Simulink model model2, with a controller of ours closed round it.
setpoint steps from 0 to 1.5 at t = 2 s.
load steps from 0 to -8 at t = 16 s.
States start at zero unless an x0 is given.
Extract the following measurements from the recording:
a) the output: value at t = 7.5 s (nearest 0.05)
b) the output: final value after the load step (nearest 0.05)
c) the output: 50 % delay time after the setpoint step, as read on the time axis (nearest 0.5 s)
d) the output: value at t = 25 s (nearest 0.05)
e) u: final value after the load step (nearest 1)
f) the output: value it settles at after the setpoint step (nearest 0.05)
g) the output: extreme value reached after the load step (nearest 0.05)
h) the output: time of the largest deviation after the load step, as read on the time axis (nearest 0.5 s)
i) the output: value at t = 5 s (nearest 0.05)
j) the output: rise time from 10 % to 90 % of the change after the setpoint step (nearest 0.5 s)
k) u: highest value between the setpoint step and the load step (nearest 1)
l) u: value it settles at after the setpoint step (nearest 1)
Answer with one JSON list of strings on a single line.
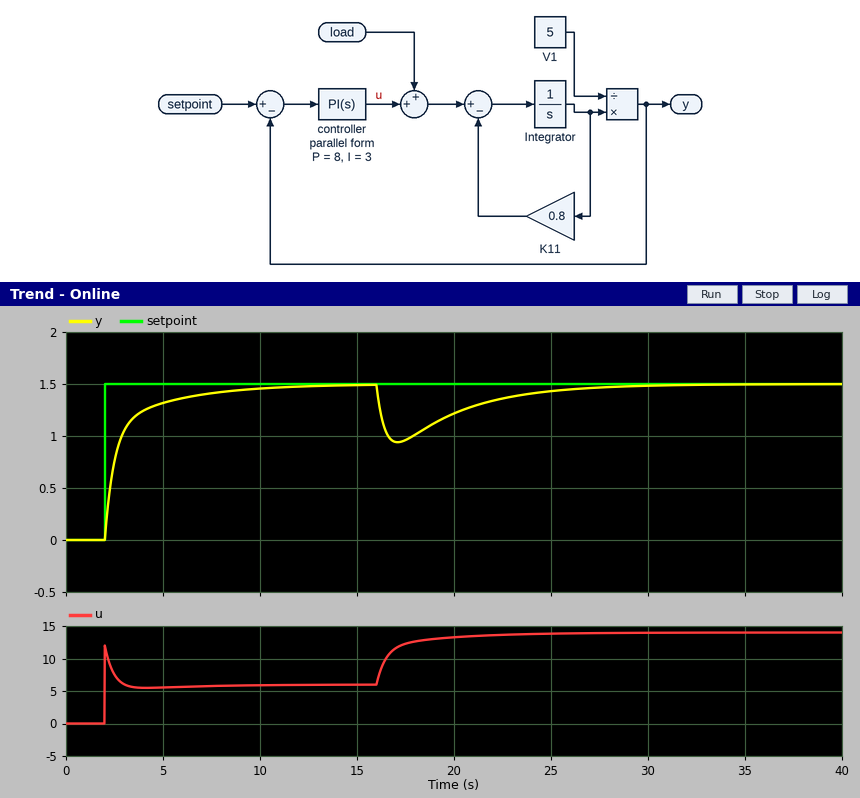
["1.40", "1.50", "2.5 s", "1.45", "14", "1.50", "0.95", "17.0 s", "1.30", "3.5 s", "12", "6"]
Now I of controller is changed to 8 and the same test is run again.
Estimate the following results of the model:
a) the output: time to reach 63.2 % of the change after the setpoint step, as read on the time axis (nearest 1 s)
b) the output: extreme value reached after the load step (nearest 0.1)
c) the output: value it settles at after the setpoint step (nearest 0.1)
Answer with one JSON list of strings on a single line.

["3 s", "1.0", "1.5"]
